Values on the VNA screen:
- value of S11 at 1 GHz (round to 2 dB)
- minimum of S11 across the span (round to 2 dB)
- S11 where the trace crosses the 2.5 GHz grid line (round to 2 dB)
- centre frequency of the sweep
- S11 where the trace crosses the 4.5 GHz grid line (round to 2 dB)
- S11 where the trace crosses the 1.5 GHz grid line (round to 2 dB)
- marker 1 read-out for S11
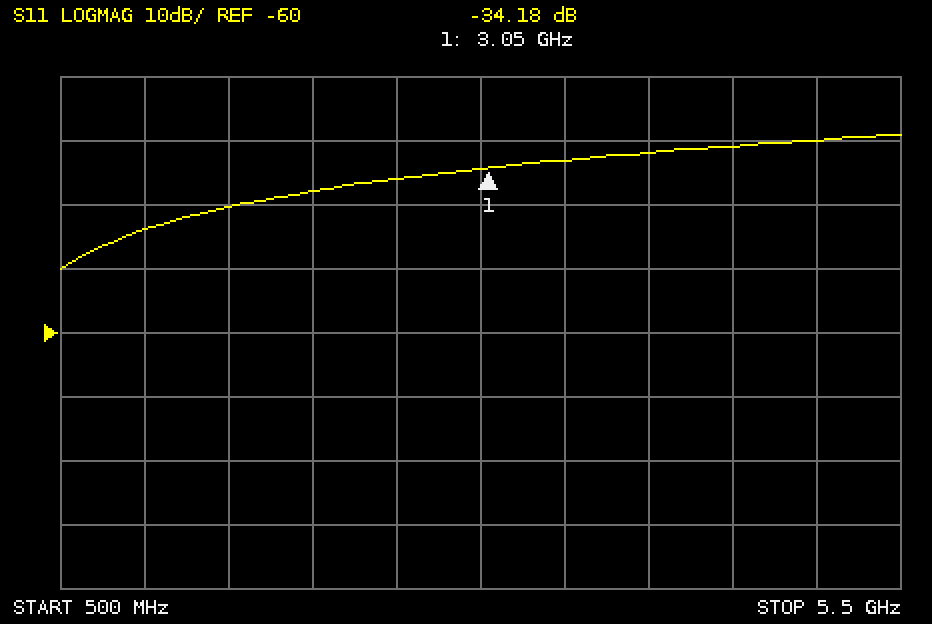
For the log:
-44 dB
-50 dB
-36 dB
3 GHz
-30 dB
-40 dB
-34.18 dB
